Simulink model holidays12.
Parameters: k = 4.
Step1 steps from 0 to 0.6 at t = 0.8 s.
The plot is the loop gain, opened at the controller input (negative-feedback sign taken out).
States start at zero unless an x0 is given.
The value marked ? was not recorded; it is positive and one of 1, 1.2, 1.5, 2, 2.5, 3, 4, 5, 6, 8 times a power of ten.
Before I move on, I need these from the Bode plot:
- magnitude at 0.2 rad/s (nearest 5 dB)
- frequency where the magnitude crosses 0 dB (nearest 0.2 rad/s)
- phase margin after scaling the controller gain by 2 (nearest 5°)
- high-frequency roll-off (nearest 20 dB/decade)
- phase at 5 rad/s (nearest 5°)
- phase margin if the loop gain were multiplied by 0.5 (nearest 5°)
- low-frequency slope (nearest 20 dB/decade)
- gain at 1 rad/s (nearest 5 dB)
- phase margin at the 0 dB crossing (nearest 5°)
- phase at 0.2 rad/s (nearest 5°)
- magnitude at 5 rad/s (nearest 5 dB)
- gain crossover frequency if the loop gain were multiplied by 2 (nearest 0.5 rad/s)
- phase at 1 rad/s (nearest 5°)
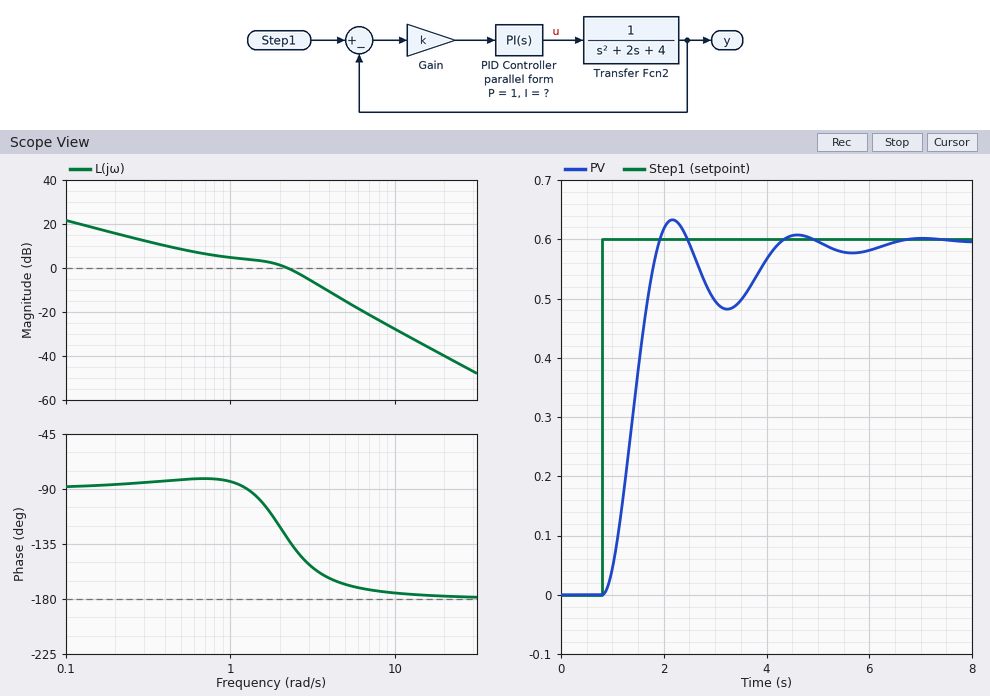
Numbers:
15 dB
2.2 rad/s
25°
-40 dB/decade
-170°
100°
-20 dB/decade
5 dB
50°
-85°
-15 dB
3.0 rad/s
-85°
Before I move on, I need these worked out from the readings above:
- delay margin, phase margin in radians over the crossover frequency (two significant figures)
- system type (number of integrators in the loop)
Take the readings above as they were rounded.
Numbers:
0.40 s
1
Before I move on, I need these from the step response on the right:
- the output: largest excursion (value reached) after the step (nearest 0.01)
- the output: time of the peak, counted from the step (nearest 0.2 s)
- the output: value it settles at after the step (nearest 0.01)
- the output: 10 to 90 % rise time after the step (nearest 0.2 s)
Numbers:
0.63
1.4 s
0.60
0.8 s
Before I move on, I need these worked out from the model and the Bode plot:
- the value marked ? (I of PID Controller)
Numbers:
1.2
